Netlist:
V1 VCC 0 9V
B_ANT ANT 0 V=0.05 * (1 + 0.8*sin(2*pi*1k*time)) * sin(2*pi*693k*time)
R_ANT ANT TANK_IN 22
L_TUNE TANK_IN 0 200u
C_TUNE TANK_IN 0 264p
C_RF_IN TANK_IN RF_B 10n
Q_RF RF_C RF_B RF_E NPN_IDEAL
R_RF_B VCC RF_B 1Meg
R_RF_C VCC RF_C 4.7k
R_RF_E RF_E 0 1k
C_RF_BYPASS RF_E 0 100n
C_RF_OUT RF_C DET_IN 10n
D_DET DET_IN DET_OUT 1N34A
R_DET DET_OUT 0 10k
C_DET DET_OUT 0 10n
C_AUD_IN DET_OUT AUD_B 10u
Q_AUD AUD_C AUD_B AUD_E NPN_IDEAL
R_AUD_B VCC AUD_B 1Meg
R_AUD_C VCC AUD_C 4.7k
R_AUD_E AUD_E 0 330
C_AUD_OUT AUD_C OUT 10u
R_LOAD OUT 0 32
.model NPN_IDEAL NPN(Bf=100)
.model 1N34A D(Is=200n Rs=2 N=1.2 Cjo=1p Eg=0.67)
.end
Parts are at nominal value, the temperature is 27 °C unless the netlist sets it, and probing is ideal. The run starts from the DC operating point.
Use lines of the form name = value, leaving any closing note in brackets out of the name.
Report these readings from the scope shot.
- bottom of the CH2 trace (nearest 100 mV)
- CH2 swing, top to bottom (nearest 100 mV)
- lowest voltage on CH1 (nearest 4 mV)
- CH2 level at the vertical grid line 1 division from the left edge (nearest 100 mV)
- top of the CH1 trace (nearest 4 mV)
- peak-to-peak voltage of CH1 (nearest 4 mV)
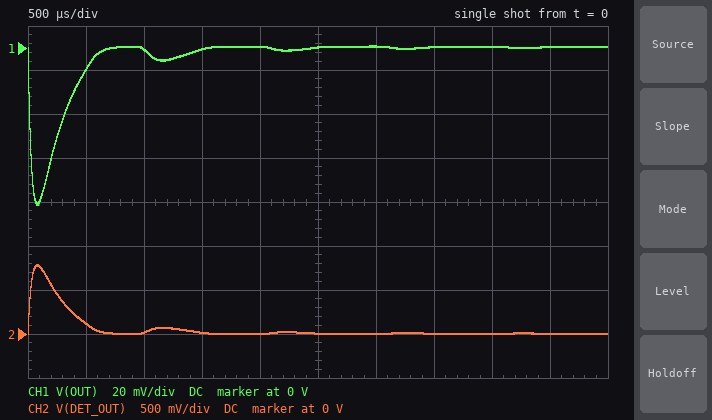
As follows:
bottom of the CH2 trace = 0 V
CH2 swing, top to bottom = 800 mV
lowest voltage on CH1 = -72 mV
CH2 level at the vertical grid line 1 division from the left edge = 100 mV
top of the CH1 trace = 0 V
peak-to-peak voltage of CH1 = 72 mV
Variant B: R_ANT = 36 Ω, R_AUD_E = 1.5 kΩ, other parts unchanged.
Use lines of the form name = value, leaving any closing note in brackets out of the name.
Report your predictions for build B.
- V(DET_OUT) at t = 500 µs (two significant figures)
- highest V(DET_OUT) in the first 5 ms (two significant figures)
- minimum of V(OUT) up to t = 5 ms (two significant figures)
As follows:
V(DET_OUT) at t = 500 µs = 170 mV
highest V(DET_OUT) in the first 5 ms = 840 mV
minimum of V(OUT) up to t = 5 ms = -17 mV
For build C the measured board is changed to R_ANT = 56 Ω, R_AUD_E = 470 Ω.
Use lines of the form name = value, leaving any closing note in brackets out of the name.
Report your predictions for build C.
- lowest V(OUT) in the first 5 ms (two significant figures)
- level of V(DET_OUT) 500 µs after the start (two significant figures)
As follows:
lowest V(OUT) in the first 5 ms = -51 mV
level of V(DET_OUT) 500 µs after the start = 130 mV
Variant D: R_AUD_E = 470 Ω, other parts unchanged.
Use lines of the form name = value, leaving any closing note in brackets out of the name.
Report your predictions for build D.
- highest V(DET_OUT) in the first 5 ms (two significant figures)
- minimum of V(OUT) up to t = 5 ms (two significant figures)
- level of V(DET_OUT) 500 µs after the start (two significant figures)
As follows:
highest V(DET_OUT) in the first 5 ms = 800 mV
minimum of V(OUT) up to t = 5 ms = -52 mV
level of V(DET_OUT) 500 µs after the start = 130 mV
